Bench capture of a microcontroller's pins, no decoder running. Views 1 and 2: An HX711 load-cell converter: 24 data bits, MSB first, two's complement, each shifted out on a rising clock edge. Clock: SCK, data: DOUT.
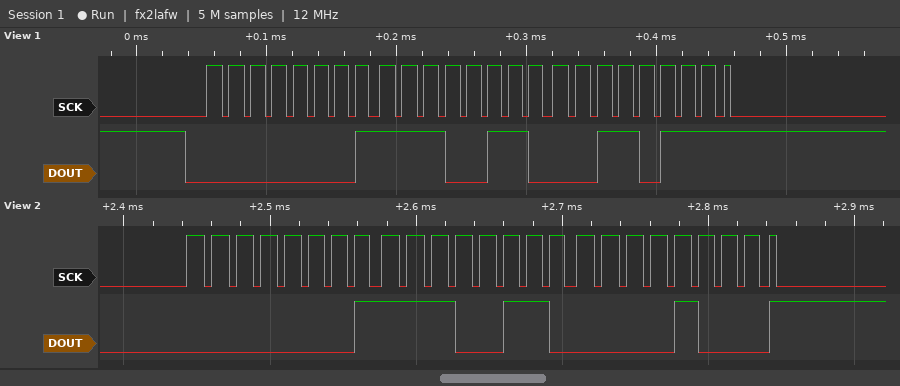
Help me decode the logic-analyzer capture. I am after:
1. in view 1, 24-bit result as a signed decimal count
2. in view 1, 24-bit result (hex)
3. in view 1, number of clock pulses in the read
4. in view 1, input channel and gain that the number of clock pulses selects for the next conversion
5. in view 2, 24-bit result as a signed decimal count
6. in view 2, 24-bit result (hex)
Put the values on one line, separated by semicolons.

124471; 0x01E637; 25; channel A, gain 128; 124424; 0x01E608
